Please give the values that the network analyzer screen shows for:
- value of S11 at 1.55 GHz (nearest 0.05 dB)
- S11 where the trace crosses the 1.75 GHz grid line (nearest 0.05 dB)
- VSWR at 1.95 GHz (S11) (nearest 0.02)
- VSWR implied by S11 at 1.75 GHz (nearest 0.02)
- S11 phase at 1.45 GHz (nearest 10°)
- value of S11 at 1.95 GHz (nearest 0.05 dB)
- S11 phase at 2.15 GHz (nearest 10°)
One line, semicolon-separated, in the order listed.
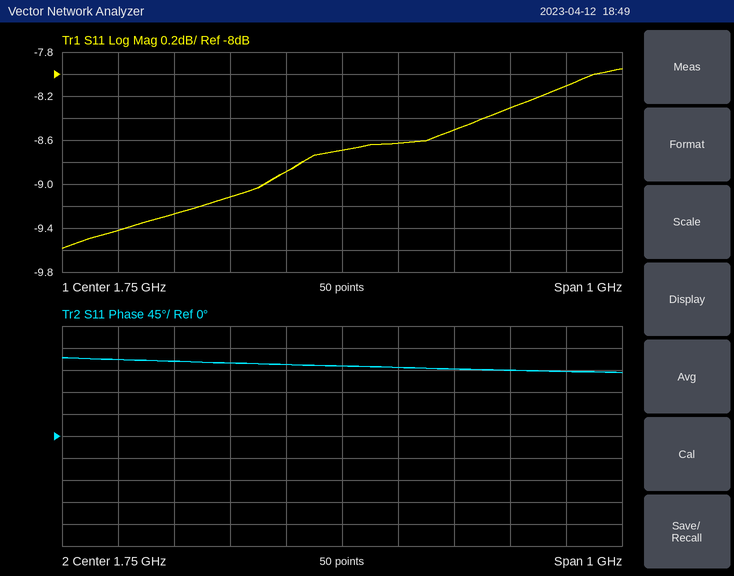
-9.10 dB; -8.70 dB; 2.20; 2.16; 150°; -8.50 dB; 130°
